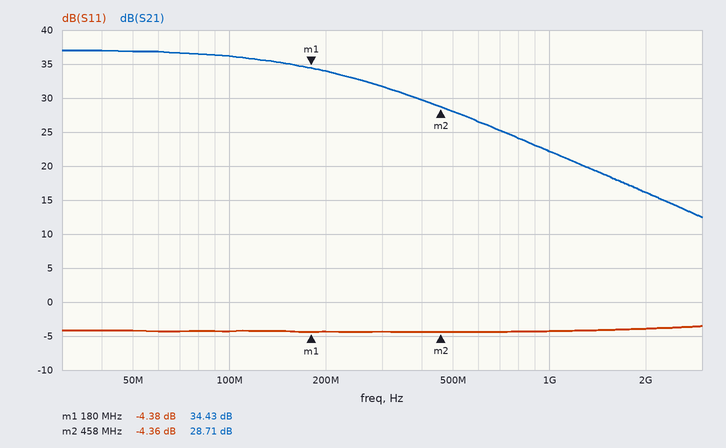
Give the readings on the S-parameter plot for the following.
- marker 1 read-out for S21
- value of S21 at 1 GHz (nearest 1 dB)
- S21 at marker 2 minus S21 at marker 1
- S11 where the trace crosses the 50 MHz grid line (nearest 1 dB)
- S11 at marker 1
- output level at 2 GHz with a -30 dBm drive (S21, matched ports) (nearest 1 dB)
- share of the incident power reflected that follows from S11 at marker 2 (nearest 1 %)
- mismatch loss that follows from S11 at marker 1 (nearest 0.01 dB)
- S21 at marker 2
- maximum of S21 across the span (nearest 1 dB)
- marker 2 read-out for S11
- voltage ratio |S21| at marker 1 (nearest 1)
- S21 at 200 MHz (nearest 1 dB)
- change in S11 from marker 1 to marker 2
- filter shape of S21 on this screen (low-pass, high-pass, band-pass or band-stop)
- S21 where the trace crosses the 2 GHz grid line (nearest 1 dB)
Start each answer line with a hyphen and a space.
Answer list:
- 34.43 dB
- 22 dB
- -5.72 dB
- -4 dB
- -4.38 dB
- -14 dBm
- 37 %
- 1.97 dB
- 28.71 dB
- 37 dB
- -4.36 dB
- 53
- 34 dB
- 0.02 dB
- low-pass
- 16 dB
